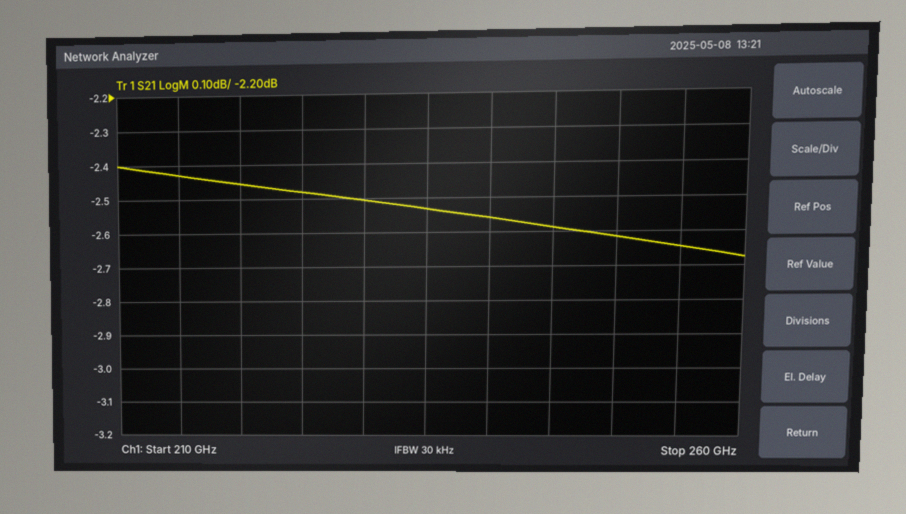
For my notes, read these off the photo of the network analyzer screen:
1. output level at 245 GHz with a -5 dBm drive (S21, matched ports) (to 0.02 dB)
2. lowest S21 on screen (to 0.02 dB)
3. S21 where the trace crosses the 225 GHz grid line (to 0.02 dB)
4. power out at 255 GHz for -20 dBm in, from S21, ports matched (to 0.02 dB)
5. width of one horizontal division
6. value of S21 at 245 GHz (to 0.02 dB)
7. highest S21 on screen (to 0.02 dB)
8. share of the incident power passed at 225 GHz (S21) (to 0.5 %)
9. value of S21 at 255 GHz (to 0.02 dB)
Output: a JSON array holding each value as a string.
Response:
["-7.58 dBm", "-2.68 dB", "-2.48 dB", "-22.64 dBm", "5 GHz", "-2.58 dB", "-2.40 dB", "56.5 %", "-2.64 dB"]
